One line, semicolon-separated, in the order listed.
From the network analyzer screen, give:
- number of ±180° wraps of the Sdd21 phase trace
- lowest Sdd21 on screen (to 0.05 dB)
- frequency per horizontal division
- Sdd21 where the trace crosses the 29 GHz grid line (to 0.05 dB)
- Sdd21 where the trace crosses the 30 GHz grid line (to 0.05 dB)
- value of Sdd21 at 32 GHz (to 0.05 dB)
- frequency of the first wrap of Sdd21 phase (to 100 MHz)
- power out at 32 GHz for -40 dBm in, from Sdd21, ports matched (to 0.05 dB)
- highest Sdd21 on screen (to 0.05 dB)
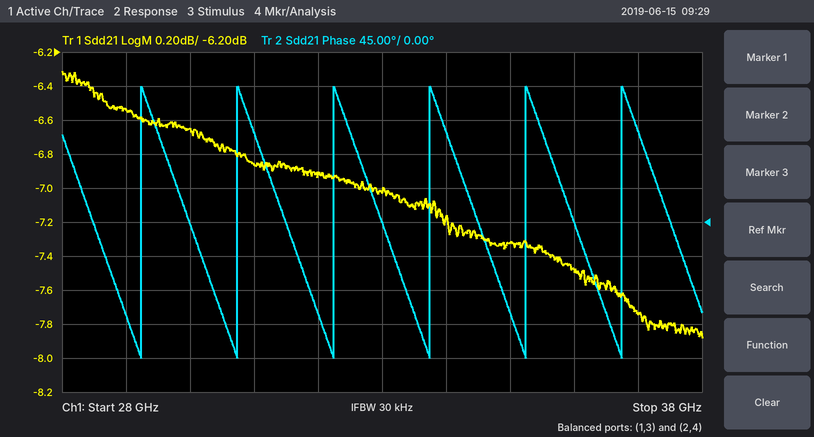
6; -7.90 dB; 1 GHz; -6.55 dB; -6.65 dB; -6.90 dB; 29.2 GHz; -46.90 dBm; -6.30 dB
